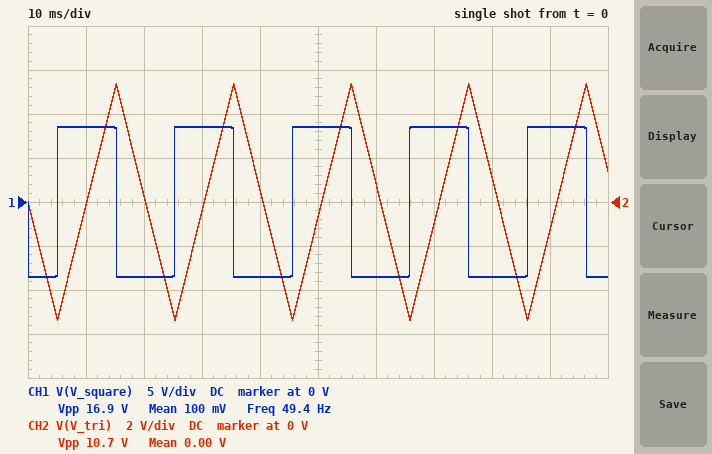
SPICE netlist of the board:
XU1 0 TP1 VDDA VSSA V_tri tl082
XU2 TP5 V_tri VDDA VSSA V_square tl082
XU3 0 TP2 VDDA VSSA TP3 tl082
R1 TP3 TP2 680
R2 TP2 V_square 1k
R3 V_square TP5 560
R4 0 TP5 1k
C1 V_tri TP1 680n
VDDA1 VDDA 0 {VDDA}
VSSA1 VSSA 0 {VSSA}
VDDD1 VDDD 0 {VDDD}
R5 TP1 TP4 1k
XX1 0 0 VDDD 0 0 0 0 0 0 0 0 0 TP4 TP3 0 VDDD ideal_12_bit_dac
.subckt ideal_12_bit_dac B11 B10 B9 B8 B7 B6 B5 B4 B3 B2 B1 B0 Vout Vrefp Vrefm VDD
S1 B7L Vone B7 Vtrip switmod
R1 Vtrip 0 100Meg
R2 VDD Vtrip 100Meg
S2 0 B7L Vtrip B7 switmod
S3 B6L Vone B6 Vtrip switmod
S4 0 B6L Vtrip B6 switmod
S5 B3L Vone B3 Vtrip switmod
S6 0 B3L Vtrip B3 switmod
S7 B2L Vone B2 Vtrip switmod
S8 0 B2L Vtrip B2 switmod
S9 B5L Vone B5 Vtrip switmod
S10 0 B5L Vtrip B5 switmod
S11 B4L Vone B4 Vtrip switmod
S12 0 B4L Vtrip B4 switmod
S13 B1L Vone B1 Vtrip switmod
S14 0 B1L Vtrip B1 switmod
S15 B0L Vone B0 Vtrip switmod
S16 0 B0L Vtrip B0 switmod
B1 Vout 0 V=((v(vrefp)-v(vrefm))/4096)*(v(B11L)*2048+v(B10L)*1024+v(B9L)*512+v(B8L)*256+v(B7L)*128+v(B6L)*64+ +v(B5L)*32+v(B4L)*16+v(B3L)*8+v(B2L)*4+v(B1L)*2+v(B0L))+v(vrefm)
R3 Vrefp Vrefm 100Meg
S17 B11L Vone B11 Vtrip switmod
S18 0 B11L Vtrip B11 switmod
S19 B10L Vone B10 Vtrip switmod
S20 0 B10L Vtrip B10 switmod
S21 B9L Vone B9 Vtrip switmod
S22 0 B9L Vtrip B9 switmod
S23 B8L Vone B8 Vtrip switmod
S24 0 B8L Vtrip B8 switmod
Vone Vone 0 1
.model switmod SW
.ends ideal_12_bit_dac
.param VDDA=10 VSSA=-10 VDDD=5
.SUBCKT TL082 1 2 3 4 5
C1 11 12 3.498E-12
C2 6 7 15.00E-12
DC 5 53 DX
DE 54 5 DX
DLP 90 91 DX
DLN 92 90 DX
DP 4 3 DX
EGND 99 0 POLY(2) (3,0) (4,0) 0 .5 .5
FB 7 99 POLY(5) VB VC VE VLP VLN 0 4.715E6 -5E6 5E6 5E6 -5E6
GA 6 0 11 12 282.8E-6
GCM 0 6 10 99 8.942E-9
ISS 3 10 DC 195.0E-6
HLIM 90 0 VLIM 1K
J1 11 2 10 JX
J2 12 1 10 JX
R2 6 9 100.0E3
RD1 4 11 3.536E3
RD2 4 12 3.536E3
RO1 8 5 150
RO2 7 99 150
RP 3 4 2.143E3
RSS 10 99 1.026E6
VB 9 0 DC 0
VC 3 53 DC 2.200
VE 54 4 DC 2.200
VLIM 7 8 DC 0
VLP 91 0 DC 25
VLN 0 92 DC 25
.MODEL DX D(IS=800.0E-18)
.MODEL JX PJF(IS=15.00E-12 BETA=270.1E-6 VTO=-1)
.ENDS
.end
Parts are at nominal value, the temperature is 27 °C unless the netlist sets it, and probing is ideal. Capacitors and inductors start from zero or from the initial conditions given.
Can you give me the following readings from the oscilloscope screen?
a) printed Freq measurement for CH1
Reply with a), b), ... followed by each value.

a) 49.4 Hz
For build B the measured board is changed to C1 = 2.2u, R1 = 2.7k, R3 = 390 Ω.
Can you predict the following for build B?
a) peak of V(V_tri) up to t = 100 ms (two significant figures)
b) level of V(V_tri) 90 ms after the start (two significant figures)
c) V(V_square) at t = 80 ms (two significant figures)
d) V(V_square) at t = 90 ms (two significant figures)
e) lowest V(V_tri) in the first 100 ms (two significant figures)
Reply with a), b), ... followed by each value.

a) 6.0 V
b) 4.8 V
c) 8.5 V
d) -8.5 V
e) -6.0 V
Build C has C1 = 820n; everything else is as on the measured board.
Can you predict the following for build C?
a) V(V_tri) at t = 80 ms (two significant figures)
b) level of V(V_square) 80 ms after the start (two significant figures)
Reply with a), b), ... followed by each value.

a) -4.8 V
b) 8.5 V
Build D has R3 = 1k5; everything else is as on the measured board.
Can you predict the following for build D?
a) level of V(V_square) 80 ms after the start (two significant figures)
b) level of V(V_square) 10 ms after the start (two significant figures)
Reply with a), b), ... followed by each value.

a) 8.5 V
b) -8.5 V
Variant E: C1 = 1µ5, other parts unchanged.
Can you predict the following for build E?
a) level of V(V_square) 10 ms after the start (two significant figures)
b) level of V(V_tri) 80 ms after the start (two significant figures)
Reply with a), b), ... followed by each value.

a) -8.5 V
b) 4.5 V
